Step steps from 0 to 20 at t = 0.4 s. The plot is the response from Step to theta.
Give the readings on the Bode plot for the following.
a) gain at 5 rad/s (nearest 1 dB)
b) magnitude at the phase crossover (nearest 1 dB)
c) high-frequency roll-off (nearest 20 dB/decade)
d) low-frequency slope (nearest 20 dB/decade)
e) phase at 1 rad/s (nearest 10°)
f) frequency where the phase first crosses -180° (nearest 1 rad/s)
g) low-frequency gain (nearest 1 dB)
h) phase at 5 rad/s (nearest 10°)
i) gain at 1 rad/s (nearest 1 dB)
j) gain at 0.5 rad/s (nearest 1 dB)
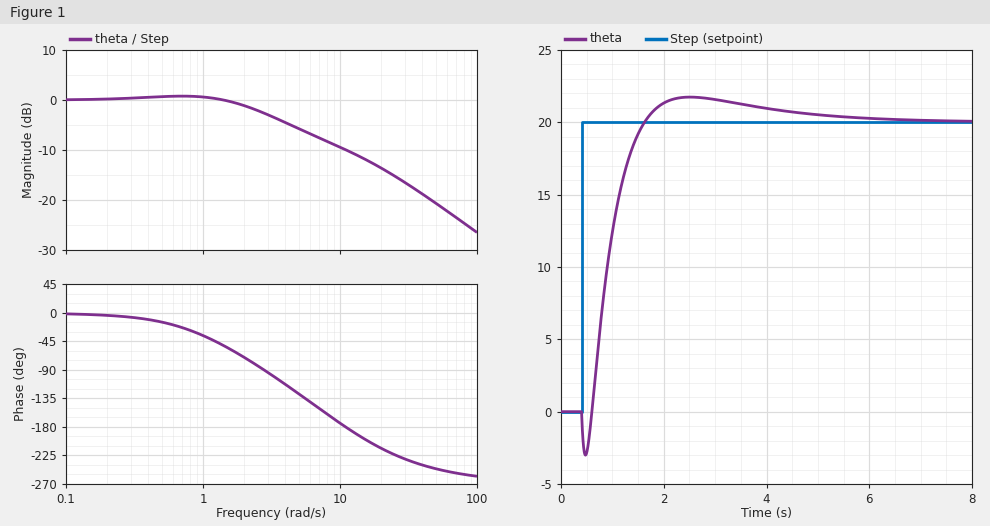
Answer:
-6 dB
-10 dB
-20 dB/decade
0 dB/decade
-40°
11 rad/s
0 dB
-130°
1 dB
1 dB
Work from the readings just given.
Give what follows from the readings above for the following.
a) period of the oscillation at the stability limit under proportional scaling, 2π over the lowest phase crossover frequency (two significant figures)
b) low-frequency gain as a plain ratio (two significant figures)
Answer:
0.57 s
1.0
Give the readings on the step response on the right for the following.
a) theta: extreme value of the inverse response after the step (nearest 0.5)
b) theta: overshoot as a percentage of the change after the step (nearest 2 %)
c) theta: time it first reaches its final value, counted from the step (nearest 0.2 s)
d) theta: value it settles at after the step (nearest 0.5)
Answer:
-3.0
8 %
1.2 s
20.0
